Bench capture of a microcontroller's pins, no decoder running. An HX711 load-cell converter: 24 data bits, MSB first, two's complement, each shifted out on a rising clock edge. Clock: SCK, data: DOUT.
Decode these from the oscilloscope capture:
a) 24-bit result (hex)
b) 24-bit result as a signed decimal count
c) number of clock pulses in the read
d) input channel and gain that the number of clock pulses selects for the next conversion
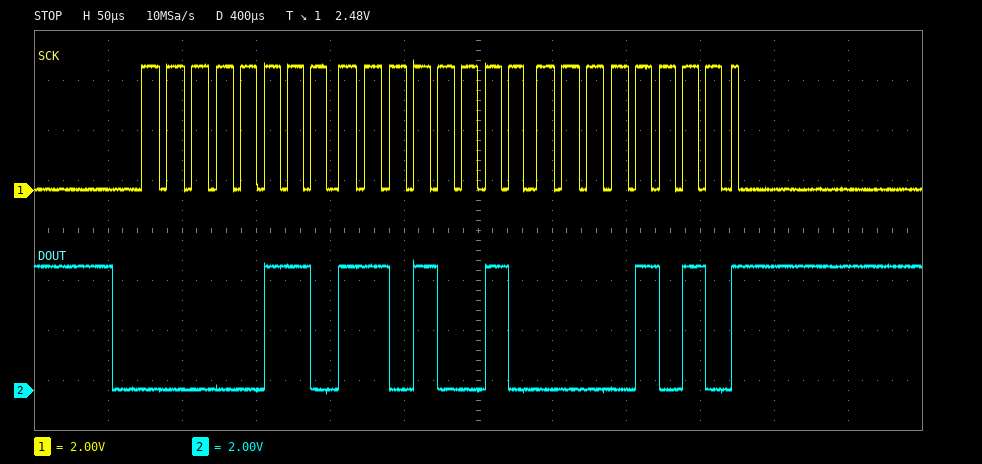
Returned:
0x06D20A
446986
25
channel A, gain 128
